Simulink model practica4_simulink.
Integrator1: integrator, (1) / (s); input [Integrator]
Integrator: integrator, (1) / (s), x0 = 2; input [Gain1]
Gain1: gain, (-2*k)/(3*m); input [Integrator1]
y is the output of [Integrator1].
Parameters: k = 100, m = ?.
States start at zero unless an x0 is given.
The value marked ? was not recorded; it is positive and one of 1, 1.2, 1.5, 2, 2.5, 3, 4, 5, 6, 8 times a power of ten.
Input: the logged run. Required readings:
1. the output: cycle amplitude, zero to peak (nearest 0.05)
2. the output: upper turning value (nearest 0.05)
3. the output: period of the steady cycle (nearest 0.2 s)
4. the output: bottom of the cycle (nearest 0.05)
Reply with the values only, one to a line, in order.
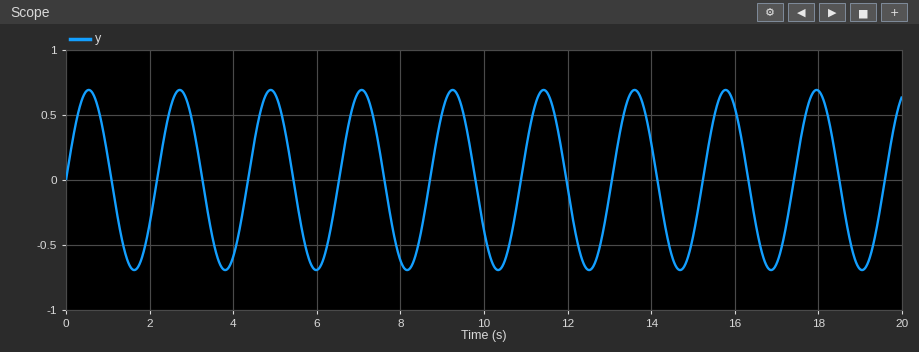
0.70
0.70
2.2 s
-0.70
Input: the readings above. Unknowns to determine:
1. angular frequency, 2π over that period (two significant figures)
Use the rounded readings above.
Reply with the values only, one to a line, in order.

2.9 rad/s
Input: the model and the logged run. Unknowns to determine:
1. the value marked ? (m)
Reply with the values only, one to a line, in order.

8
